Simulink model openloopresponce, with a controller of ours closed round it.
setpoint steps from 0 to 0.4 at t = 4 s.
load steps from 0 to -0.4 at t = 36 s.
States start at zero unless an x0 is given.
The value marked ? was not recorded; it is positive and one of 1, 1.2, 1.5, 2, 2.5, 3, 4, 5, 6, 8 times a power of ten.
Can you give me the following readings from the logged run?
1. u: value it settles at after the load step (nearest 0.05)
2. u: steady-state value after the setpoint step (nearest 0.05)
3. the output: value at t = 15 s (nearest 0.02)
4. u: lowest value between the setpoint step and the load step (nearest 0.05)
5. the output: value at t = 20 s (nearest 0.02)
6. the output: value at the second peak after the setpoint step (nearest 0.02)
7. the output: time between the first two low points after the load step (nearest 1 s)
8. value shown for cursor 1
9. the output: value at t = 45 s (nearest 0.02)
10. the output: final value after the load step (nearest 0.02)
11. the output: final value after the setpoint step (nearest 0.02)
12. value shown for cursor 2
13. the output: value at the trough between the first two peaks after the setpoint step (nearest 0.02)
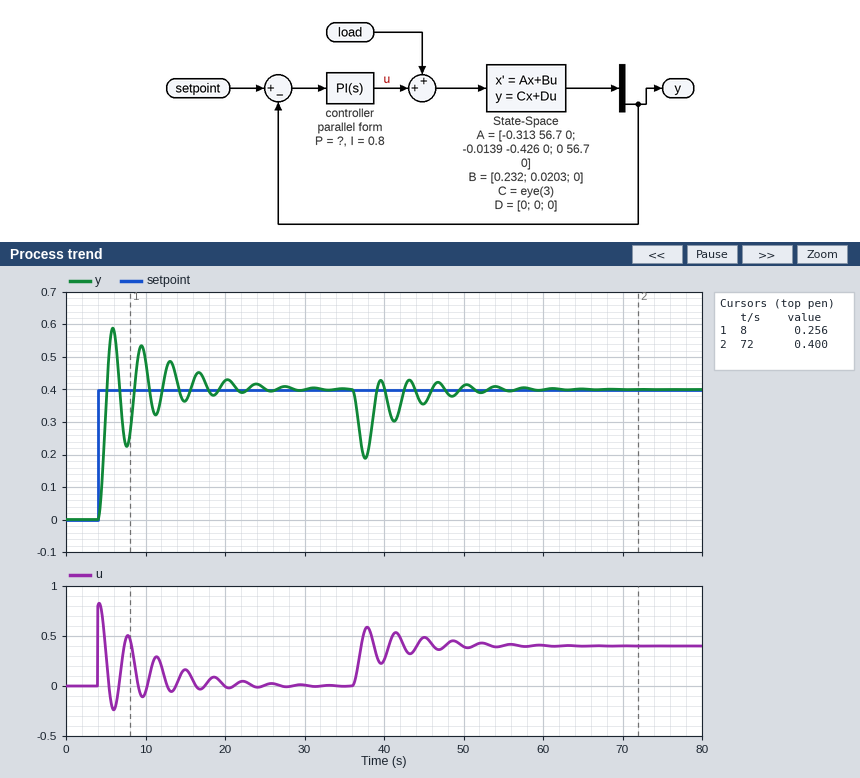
0.40
0.00
0.36
-0.25
0.42
0.54
4 s
0.256
0.36
0.40
0.40
0.400
0.22
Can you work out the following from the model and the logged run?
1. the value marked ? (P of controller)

2
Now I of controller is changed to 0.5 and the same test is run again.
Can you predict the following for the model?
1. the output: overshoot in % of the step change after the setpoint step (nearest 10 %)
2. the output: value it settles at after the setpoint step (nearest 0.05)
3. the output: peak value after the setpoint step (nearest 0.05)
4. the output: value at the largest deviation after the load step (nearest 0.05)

40 %
0.40
0.55
0.20
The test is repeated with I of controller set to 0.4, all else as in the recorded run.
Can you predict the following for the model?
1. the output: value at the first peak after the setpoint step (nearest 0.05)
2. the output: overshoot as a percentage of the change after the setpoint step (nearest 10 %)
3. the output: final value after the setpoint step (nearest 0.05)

0.55
30 %
0.40
